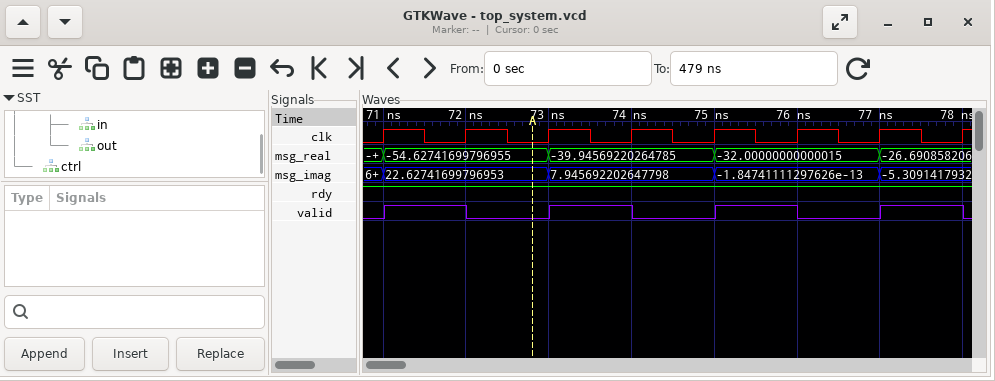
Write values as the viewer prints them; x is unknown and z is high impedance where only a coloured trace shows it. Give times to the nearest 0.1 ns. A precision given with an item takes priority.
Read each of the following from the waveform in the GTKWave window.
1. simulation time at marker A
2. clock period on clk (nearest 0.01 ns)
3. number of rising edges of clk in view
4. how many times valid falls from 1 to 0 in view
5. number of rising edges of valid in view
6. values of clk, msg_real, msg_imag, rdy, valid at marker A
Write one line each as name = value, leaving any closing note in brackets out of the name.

simulation time at marker A = 72.8 ns
clock period on clk = 1 ns
number of rising edges of clk in view = 8
how many times valid falls from 1 to 0 in view = 4
number of rising edges of valid in view = 4
values of clk, msg_real, msg_imag, rdy, valid at marker A = clk=0, msg_real=-54.62741699796955, msg_imag=22.62741699796953, rdy=1, valid=0
